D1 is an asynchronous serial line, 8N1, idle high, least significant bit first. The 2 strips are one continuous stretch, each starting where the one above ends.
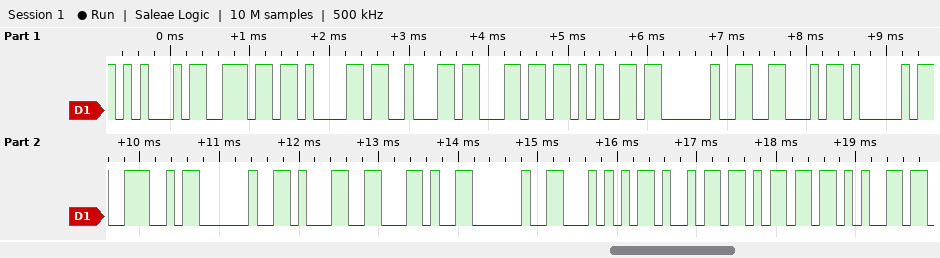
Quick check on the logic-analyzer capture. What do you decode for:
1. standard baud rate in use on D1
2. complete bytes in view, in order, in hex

9600 baud
0x45 0x6E 0x61 0x62 0x6C 0x65 0x20 0x46 0x41 0x4E 0x20 0x31 0x2C 0x20 0x54 0x69 0x6D 0x65
